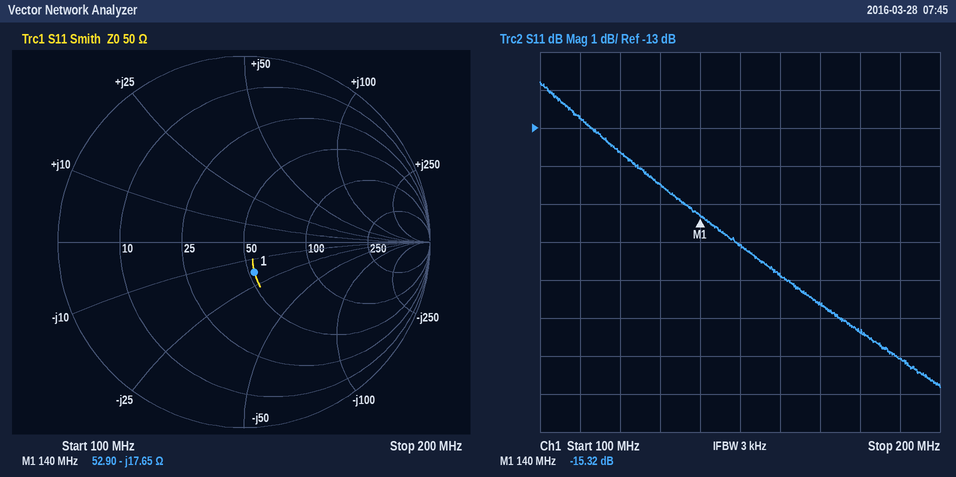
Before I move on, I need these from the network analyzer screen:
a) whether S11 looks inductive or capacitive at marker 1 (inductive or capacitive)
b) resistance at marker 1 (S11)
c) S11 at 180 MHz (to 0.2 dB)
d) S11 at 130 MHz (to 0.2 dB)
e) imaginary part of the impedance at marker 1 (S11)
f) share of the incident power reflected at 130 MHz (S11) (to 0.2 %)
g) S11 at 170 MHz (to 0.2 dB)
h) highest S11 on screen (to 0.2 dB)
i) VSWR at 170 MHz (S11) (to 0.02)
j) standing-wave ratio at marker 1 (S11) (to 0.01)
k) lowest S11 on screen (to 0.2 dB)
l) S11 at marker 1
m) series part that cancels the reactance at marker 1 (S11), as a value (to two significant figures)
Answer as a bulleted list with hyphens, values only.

- capacitive
- 52.90 Ω
- -18.4 dB
- -14.4 dB
- -17.65 Ω
- 3.6 %
- -17.6 dB
- -11.8 dB
- 1.30
- 1.41
- -19.8 dB
- -15.32 dB
- 20 nH
